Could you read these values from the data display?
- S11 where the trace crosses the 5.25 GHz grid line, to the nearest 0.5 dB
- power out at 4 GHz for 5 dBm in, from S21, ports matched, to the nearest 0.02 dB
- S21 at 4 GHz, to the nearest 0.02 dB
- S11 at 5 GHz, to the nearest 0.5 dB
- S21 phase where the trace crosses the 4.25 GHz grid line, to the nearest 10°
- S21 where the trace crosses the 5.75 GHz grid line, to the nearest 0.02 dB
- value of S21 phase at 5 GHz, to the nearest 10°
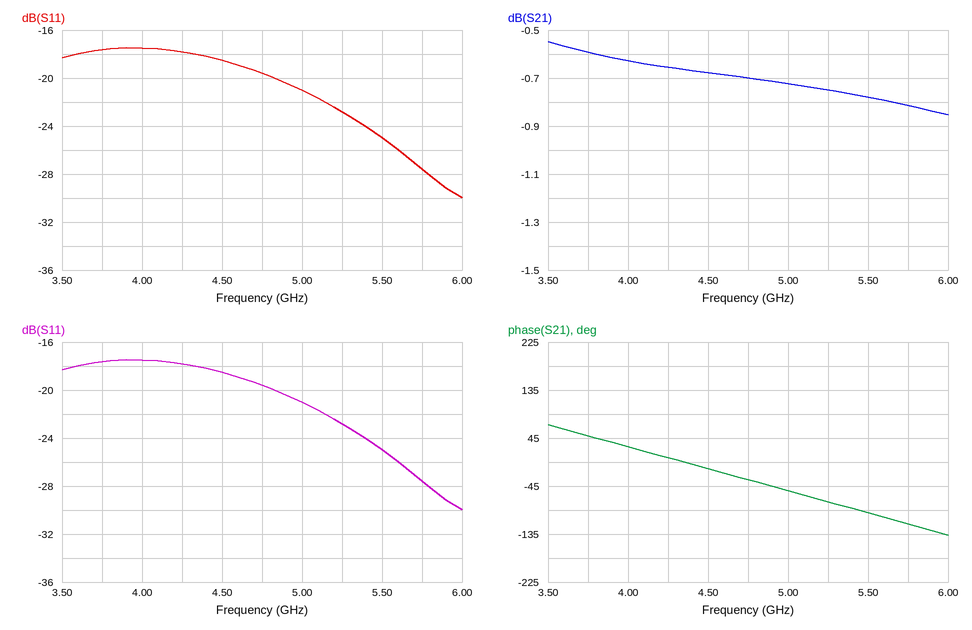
-23.0 dB
4.38 dBm
-0.62 dB
-21.0 dB
10°
-0.82 dB
-50°
